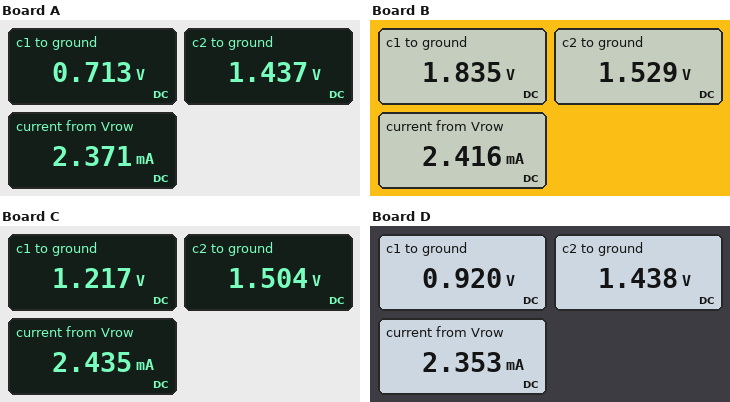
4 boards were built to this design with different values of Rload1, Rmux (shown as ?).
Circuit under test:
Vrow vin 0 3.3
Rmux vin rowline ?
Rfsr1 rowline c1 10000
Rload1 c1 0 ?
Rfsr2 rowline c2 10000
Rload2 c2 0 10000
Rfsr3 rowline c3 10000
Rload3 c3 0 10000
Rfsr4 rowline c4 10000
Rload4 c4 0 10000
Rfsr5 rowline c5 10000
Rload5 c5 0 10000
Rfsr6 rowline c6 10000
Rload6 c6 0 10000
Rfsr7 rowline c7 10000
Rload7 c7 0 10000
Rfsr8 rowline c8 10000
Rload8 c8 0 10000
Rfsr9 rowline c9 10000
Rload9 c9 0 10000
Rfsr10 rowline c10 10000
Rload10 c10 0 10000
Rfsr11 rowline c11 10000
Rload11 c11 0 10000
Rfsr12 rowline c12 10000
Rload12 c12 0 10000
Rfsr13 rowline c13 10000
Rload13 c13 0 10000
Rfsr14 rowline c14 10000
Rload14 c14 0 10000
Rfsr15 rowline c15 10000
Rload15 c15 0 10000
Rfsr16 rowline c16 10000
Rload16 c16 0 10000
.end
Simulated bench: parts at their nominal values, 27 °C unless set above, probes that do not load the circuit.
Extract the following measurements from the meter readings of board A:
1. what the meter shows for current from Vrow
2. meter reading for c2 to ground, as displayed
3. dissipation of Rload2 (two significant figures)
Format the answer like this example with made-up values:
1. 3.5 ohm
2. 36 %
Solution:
1. 2.371 mA
2. 1.437 V
3. 210 µW
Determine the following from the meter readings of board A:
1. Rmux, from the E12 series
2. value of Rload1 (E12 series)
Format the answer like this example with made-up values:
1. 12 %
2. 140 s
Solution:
1. 180 Ω
2. 3.3 kΩ
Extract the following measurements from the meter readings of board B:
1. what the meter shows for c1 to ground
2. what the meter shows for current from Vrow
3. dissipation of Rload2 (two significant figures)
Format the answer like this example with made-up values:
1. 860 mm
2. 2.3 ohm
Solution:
1. 1.835 V
2. 2.416 mA
3. 230 µW
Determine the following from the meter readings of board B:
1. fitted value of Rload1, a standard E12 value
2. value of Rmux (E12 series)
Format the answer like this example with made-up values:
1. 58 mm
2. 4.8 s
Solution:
1. 15 kΩ
2. 100 Ω
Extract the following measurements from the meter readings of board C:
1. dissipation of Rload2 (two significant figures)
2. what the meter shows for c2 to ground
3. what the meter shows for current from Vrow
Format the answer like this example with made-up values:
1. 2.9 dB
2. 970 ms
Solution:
1. 230 µW
2. 1.504 V
3. 2.435 mA
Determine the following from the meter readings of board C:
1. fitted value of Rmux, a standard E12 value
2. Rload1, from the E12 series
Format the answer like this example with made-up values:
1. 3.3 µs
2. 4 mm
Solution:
1. 120 Ω
2. 6.8 kΩ
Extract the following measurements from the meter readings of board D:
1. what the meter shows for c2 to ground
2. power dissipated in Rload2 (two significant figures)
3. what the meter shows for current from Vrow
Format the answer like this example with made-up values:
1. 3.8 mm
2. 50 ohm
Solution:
1. 1.438 V
2. 210 µW
3. 2.353 mA
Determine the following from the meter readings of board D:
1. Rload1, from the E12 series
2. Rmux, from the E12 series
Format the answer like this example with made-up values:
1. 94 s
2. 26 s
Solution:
1. 4.7 kΩ
2. 180 Ω
